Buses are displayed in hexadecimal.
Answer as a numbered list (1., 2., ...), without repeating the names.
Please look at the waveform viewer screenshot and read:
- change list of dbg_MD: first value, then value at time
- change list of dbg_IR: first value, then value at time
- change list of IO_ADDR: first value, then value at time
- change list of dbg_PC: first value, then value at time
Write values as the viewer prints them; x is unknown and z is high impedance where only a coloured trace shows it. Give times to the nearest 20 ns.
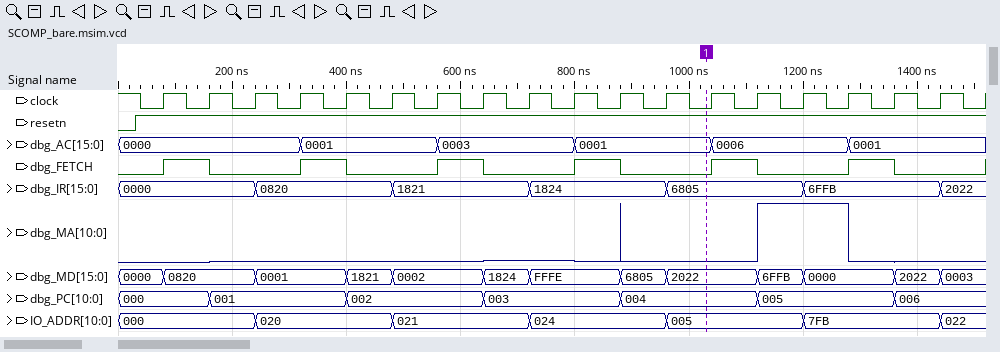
1. 0000, 0820 at 80 ns, 0001 at 240 ns, 1821 at 400 ns, 0002 at 480 ns, 1824 at 640 ns, FFFE at 720 ns, 6805 at 880 ns, 2022 at 960 ns, 6FFB at 1120 ns, 0000 at 1200 ns, 2022 at 1360 ns, 0003 at 1440 ns
2. 0000, 0820 at 240 ns, 1821 at 480 ns, 1824 at 720 ns, 6805 at 960 ns, 6FFB at 1200 ns, 2022 at 1440 ns
3. 000, 020 at 240 ns, 021 at 480 ns, 024 at 720 ns, 005 at 960 ns, 7FB at 1200 ns, 022 at 1440 ns
4. 000, 001 at 160 ns, 002 at 400 ns, 003 at 640 ns, 004 at 880 ns, 005 at 1120 ns, 006 at 1360 ns
